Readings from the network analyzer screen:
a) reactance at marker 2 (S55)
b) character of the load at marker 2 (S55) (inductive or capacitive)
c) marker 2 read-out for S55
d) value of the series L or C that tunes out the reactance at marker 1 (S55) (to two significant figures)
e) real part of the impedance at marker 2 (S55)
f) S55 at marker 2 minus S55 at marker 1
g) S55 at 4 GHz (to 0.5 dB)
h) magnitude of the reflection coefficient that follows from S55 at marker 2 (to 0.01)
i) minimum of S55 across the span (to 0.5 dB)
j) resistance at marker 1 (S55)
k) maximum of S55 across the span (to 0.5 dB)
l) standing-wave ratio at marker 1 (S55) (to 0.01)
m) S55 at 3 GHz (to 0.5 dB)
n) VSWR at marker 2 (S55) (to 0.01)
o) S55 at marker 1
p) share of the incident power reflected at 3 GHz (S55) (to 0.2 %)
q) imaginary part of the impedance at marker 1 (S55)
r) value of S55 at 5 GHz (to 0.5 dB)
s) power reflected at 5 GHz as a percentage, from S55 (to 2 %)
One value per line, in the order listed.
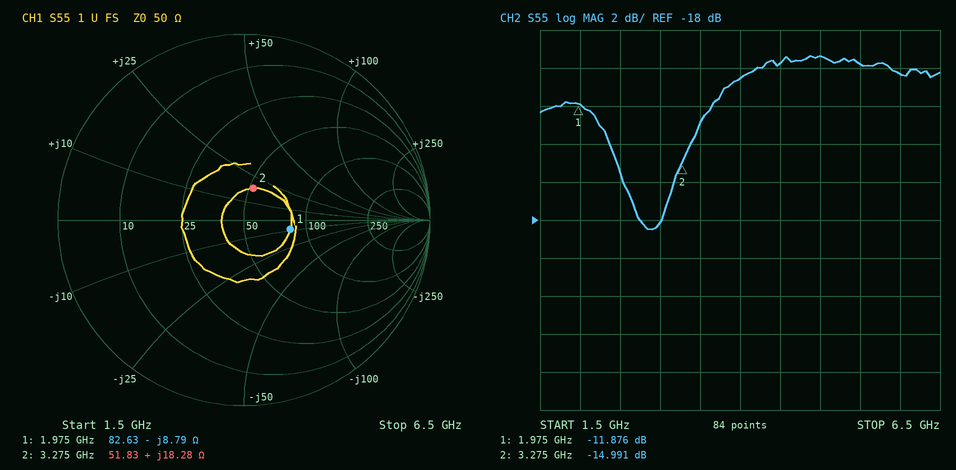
+18.28 Ω
inductive
-14.991 dB
710 pH
51.83 Ω
-3.115 dB
-10.5 dB
0.18
-18.5 dB
82.63 Ω
-9.5 dB
1.68
-18.0 dB
1.43
-11.876 dB
1.6 %
-8.79 Ω
-9.5 dB
12 %
